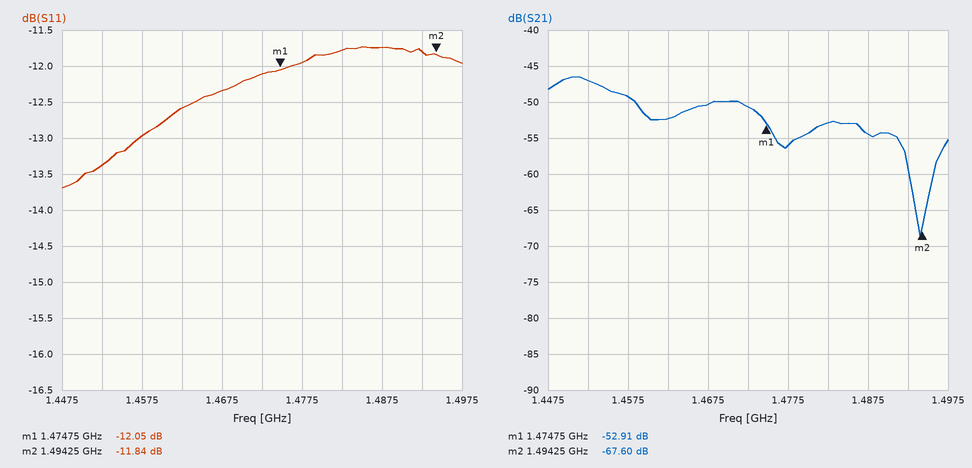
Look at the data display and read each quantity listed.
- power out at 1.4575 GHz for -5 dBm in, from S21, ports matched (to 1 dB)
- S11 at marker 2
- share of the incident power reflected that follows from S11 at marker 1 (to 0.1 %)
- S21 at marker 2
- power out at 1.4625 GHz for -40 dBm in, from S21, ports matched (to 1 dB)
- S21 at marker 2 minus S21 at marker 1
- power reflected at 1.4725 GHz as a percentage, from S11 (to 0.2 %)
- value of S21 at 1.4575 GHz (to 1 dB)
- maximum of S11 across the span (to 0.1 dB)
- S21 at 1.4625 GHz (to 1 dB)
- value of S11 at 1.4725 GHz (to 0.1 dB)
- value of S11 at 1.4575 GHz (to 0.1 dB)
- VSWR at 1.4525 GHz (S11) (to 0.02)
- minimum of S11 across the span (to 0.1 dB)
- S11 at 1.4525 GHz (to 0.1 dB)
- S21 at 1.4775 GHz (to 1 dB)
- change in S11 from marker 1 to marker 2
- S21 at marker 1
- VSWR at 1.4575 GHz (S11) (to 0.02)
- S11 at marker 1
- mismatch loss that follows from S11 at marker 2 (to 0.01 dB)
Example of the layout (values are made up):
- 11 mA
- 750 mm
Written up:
- -54 dBm
- -11.84 dB
- 6.2 %
- -67.60 dB
- -92 dBm
- -14.69 dB
- 6.2 %
- -49 dB
- -11.7 dB
- -52 dB
- -12.1 dB
- -13.0 dB
- 1.54
- -13.7 dB
- -13.4 dB
- -56 dB
- 0.21 dB
- -52.91 dB
- 1.58
- -12.05 dB
- 0.29 dB
